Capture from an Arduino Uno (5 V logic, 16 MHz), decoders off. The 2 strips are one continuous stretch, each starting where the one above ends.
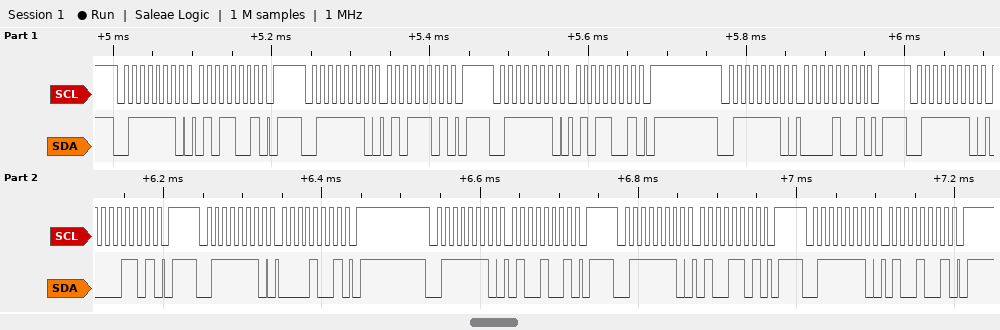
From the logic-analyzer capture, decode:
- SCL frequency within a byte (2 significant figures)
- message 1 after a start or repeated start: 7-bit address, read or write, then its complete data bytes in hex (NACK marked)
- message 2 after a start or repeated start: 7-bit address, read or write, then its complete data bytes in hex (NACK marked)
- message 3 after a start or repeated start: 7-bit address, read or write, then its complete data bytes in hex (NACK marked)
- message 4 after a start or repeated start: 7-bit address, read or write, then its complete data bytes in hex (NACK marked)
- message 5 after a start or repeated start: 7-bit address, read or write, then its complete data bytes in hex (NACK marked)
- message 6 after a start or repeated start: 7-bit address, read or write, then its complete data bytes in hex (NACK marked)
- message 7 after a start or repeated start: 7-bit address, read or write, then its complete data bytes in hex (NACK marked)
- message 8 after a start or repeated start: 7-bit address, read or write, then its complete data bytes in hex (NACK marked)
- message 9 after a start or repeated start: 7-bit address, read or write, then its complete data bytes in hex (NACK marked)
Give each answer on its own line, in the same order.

100 kHz
0x3F write: 59
0x3F write: 5D
0x3F write: 59
0x3F write: 09
0x3F write: 0D
0x3F write: 09
0x3F write: 49
0x3F write: 4D
0x3F write: 49
